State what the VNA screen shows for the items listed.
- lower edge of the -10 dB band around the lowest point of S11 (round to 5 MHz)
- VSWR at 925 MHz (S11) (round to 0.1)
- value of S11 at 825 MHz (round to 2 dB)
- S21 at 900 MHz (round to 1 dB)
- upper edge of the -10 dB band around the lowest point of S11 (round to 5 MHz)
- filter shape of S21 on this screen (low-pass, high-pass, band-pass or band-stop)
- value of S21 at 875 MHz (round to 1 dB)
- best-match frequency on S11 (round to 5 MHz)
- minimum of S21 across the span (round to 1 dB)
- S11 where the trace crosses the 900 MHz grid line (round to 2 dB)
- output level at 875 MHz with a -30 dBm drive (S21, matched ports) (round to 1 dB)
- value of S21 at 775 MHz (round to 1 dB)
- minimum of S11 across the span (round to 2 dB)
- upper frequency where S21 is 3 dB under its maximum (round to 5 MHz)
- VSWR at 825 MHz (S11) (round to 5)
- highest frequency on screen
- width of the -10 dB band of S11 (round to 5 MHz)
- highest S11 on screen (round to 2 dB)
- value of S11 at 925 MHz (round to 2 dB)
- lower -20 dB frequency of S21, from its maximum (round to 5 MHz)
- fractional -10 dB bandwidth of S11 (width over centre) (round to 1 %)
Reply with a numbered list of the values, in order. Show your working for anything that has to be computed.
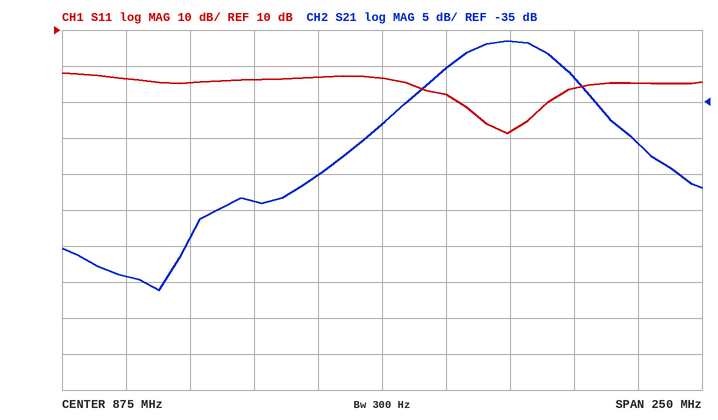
1. 905 MHz
2. |Γ| = 10^(-18/20) = 0.1259; VSWR = (1 + 0.1259)/(1 − 0.1259) ≈ 1.3
3. -4 dB
4. -30 dB
5. 940 MHz
6. band-pass
7. -38 dB
8. 925 MHz
9. -61 dB
10. -8 dB
11. -30 dBm + (-38 dB) = -68 dBm
12. -59 dB
13. -18 dB
14. 945 MHz
15. |Γ| = 10^(-4/20) = 0.6310; VSWR = (1 + 0.6310)/(1 − 0.6310) ≈ 4.42, so 5 to the nearest 5
16. 1 GHz
17. 940 MHz − 905 MHz = 35 MHz
18. -2 dB
19. -18 dB
20. 845 MHz
21. 35 MHz / 922.5 MHz ≈ 4 %
